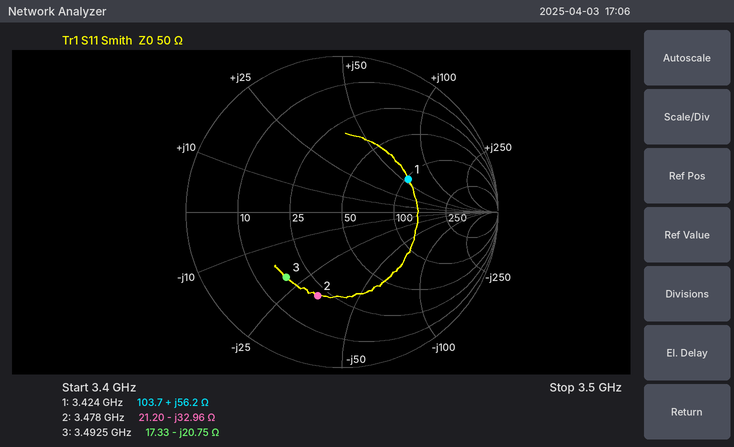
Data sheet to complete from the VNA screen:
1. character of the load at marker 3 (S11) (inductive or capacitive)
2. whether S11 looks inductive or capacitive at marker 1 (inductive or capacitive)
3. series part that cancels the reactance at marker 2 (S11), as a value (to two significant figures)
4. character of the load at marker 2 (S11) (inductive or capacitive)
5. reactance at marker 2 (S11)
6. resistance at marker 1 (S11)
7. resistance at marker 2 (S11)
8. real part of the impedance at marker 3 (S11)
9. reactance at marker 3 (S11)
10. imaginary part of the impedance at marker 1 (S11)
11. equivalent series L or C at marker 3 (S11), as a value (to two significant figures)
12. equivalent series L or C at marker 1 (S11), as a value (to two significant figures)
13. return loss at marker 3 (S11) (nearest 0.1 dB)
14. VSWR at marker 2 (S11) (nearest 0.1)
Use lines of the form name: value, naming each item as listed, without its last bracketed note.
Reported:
character of the load at marker 3 (S11): capacitive
whether S11 looks inductive or capacitive at marker 1: inductive
series part that cancels the reactance at marker 2 (S11), as a value: 1.5 nH
character of the load at marker 2 (S11): capacitive
reactance at marker 2: -32.96 Ω
resistance at marker 1: 103.7 Ω
resistance at marker 2: 21.20 Ω
real part of the impedance at marker 3: 17.33 Ω
reactance at marker 3: -20.75 Ω
imaginary part of the impedance at marker 1: +56.2 Ω
equivalent series L or C at marker 3 (S11), as a value: 2.2 pF
equivalent series L or C at marker 1 (S11), as a value: 2.6 nH
return loss at marker 3 (S11): 5.2 dB
VSWR at marker 2 (S11): 3.5
